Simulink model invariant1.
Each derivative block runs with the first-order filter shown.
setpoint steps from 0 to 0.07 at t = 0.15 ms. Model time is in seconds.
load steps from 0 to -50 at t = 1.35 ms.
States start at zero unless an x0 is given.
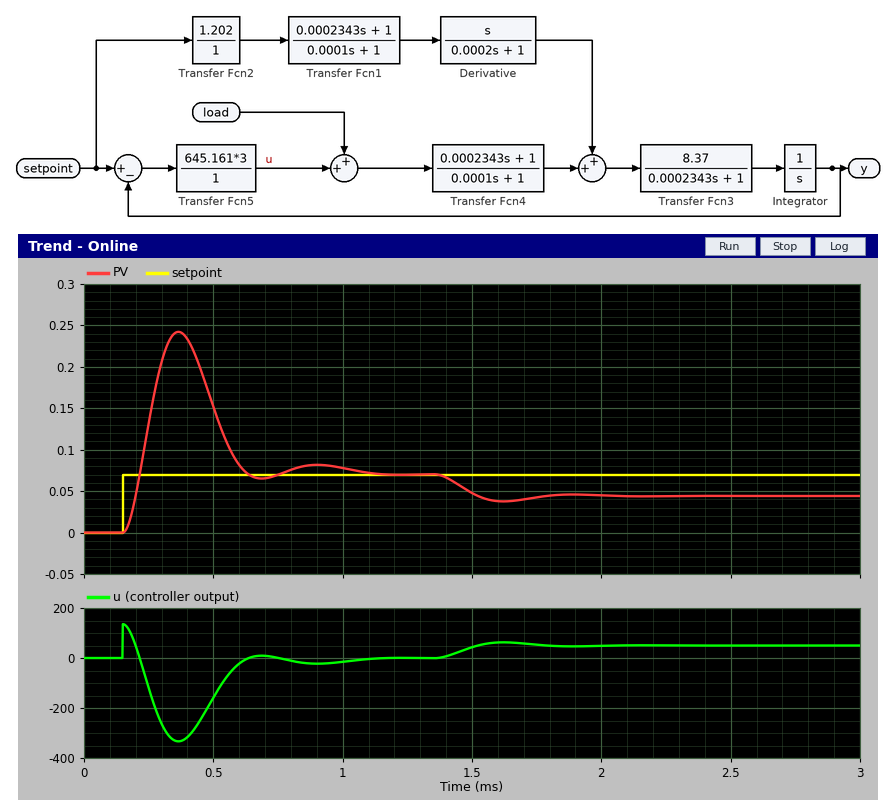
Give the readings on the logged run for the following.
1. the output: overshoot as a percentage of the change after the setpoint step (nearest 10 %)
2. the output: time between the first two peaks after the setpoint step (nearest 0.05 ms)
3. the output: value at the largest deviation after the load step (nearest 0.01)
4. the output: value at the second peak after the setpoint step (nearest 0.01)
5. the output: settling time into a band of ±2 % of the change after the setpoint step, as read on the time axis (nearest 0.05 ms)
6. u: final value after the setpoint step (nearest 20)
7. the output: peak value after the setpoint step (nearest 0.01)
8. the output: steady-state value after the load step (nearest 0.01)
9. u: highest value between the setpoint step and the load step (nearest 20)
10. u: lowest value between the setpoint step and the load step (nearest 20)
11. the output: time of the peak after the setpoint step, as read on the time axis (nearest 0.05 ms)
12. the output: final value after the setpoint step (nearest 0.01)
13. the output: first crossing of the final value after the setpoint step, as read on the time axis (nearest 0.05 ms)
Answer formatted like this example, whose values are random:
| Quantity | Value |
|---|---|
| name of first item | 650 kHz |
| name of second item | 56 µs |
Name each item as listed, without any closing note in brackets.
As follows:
| Quantity | Value |
|---|---|
| the output: overshoot as a percentage of the change after the setpoint step | 250 % |
| the output: time between the first two peaks after the setpoint step | 0.55 ms |
| the output: value at the largest deviation after the load step | 0.04 |
| the output: value at the second peak after the setpoint step | 0.08 |
| the output: settling time into a band of ±2 % of the change after the setpoint step, as read on the time axis | 1.10 ms |
| u: final value after the setpoint step | 0 |
| the output: peak value after the setpoint step | 0.24 |
| the output: steady-state value after the load step | 0.04 |
| u: highest value between the setpoint step and the load step | 140 |
| u: lowest value between the setpoint step and the load step | -340 |
| the output: time of the peak after the setpoint step, as read on the time axis | 0.35 ms |
| the output: final value after the setpoint step | 0.07 |
| the output: first crossing of the final value after the setpoint step, as read on the time axis | 0.20 ms |
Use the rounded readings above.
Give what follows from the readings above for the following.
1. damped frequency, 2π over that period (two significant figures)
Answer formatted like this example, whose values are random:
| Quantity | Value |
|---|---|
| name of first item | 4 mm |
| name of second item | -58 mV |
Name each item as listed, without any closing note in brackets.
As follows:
| Quantity | Value |
|---|---|
| damped frequency, 2π over that period | 11 rad/ms |
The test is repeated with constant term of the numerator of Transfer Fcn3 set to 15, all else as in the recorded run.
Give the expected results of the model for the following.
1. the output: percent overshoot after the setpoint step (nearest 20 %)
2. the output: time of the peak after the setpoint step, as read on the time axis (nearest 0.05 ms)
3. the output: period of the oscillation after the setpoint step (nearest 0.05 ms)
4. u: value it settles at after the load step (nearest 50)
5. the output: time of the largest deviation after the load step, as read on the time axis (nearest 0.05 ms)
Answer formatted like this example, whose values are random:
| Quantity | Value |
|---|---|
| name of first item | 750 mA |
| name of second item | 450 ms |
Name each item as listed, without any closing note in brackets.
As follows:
| Quantity | Value |
|---|---|
| the output: percent overshoot after the setpoint step | 320 % |
| the output: time of the peak after the setpoint step, as read on the time axis | 0.30 ms |
| the output: period of the oscillation after the setpoint step | 0.40 ms |
| u: value it settles at after the load step | 50 |
| the output: time of the largest deviation after the load step, as read on the time axis | 1.55 ms |
